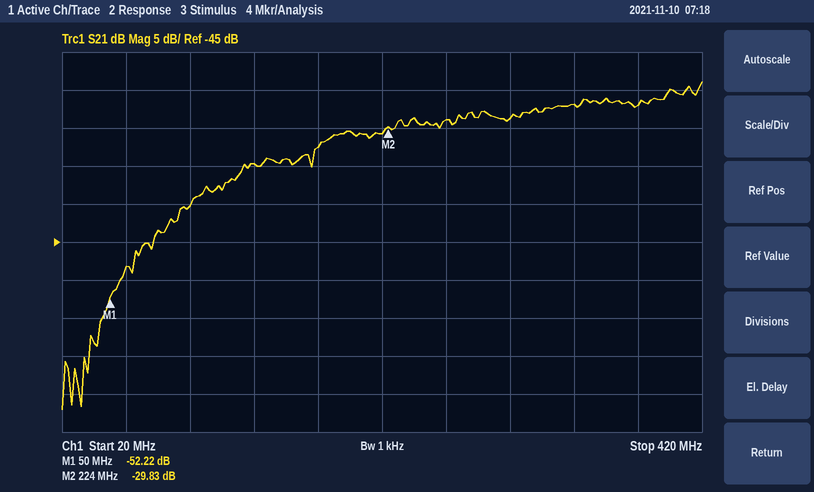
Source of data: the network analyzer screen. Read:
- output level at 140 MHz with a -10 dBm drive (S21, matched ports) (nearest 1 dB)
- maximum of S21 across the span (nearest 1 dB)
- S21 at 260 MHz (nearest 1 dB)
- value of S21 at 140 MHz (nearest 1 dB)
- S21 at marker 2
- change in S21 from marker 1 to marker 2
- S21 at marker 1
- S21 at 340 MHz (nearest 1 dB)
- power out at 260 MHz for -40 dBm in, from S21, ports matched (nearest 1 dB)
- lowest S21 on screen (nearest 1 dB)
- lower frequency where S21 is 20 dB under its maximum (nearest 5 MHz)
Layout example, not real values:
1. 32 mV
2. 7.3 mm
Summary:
1. -45 dBm
2. -24 dB
3. -29 dB
4. -35 dB
5. -29.83 dB
6. 22.39 dB
7. -52.22 dB
8. -27 dB
9. -69 dBm
10. -67 dB
11. 80 MHz
